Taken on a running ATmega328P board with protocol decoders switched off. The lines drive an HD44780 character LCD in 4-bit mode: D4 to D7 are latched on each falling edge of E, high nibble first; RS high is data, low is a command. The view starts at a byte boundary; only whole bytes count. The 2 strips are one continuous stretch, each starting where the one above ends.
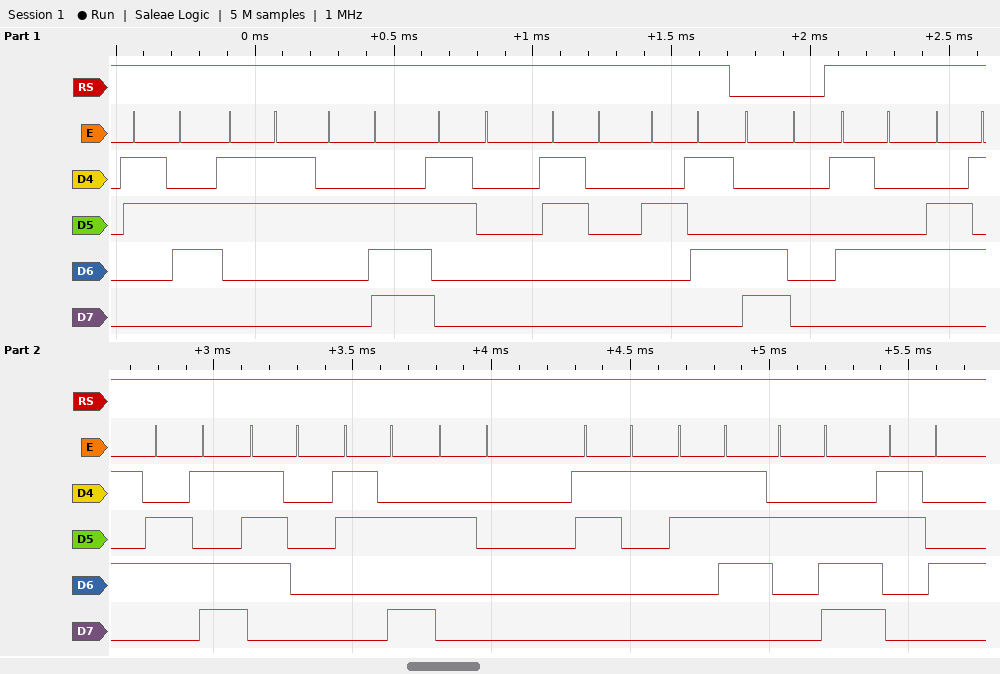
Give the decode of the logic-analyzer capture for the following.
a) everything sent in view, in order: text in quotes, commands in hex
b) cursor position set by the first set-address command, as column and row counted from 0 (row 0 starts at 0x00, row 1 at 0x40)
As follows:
"63.00%" 0xC0 "Temp: 17.4"
column 0, row 1
